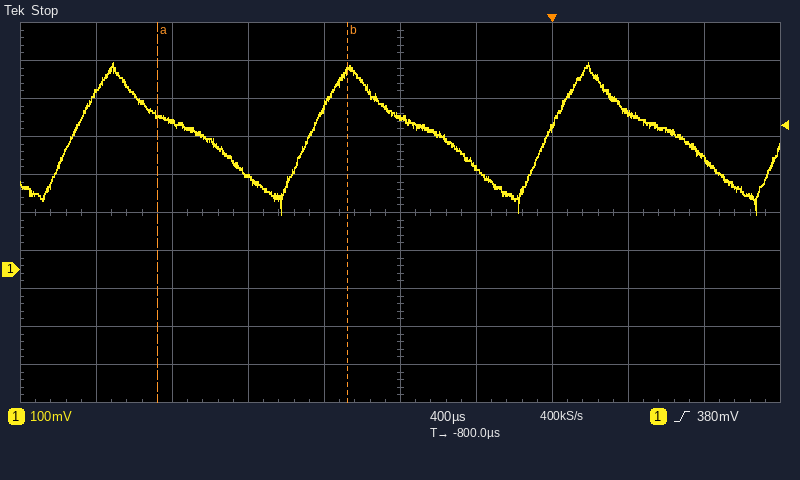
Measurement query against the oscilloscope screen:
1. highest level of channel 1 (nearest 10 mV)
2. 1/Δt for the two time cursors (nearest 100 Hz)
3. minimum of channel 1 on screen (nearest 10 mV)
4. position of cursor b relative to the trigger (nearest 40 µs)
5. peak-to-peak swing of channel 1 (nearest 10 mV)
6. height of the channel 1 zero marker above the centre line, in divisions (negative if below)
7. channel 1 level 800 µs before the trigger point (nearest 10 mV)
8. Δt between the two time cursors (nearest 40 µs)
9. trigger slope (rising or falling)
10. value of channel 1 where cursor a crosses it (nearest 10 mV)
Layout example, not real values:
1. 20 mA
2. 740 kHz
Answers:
1. 540 mV
2. 1.0 kHz
3. 140 mV
4. -1.08 ms
5. 400 mV
6. -1.5 div
7. 400 mV
8. 1.00 ms
9. rising
10. 410 mV
